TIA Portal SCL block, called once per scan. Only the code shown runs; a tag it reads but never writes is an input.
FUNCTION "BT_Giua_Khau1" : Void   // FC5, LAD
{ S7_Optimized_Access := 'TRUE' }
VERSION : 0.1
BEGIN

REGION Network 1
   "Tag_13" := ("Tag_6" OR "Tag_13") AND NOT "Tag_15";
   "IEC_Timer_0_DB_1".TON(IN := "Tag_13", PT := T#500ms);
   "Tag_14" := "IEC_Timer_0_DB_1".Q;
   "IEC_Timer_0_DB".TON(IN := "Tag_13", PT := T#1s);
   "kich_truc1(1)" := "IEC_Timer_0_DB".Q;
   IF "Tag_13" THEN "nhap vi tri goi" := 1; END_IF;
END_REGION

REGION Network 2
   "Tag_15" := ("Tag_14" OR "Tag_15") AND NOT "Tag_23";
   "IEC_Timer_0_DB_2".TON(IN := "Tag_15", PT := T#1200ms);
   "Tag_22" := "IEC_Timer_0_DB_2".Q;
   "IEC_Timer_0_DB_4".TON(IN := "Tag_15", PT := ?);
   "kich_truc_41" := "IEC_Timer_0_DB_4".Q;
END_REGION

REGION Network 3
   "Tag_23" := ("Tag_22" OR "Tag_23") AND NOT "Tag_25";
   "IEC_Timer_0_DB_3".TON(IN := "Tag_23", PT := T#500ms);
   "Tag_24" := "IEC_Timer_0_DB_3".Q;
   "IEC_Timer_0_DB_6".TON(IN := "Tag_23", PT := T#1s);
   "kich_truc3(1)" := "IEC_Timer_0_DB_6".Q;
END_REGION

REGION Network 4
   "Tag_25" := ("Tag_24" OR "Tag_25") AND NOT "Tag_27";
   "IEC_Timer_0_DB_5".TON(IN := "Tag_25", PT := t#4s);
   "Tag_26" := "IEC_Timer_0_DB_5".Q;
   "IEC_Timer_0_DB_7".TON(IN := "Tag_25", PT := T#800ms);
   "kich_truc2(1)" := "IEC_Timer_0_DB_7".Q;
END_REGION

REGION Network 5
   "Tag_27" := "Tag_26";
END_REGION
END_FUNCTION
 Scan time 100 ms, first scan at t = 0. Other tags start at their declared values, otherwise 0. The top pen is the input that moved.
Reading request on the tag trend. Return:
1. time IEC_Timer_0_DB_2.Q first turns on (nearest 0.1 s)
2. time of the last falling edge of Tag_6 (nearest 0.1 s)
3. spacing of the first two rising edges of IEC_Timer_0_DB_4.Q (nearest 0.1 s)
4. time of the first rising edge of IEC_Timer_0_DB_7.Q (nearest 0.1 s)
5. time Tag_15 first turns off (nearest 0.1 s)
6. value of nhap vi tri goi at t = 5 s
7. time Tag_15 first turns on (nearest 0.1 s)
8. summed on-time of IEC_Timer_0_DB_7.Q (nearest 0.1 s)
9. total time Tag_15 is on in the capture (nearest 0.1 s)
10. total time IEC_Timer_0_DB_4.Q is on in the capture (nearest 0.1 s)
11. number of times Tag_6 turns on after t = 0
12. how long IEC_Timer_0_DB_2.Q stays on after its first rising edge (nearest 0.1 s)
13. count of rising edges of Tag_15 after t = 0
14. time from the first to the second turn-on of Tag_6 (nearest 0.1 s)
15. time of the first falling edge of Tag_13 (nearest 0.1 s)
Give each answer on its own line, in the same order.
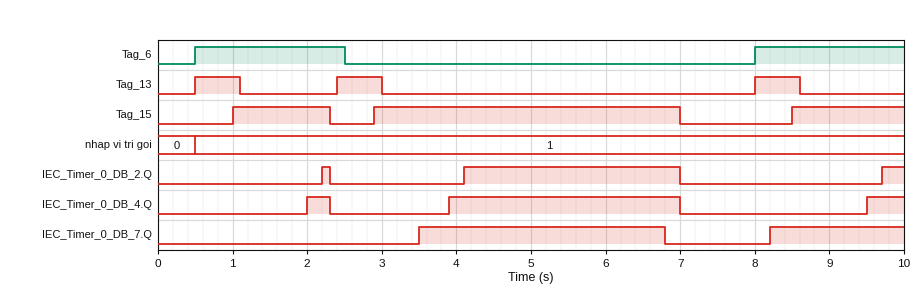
2.2 s
2.5 s
1.9 s
3.5 s
2.3 s
1
1.0 s
5.1 s
6.9 s
3.9 s
2
0.1 s
3
7.5 s
1.1 s
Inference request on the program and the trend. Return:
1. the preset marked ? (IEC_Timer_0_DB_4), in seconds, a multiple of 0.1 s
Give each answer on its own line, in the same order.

1.0 s
